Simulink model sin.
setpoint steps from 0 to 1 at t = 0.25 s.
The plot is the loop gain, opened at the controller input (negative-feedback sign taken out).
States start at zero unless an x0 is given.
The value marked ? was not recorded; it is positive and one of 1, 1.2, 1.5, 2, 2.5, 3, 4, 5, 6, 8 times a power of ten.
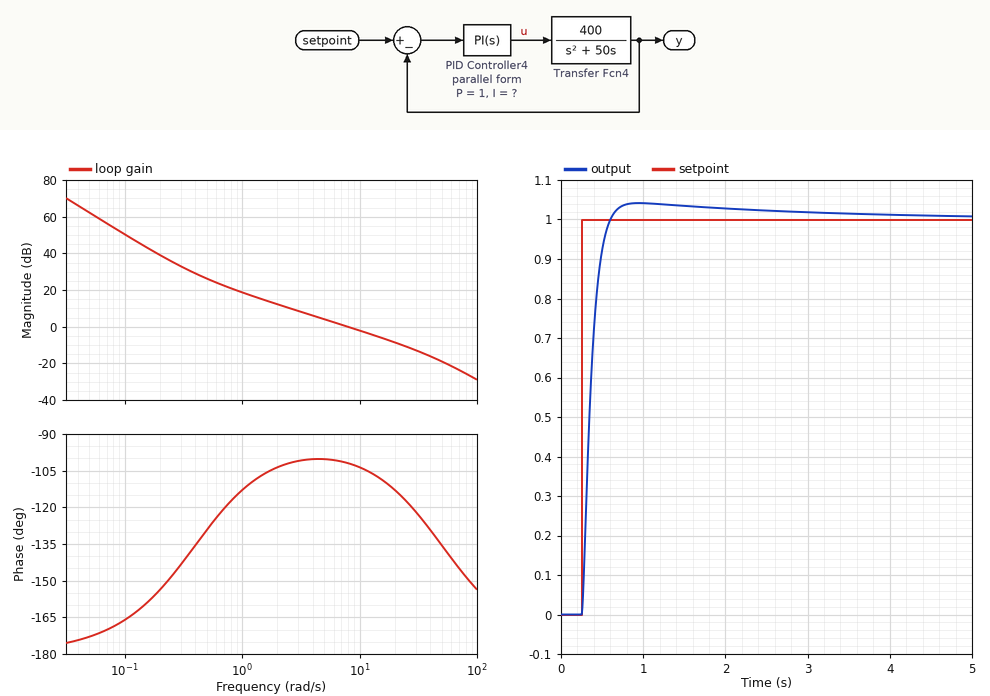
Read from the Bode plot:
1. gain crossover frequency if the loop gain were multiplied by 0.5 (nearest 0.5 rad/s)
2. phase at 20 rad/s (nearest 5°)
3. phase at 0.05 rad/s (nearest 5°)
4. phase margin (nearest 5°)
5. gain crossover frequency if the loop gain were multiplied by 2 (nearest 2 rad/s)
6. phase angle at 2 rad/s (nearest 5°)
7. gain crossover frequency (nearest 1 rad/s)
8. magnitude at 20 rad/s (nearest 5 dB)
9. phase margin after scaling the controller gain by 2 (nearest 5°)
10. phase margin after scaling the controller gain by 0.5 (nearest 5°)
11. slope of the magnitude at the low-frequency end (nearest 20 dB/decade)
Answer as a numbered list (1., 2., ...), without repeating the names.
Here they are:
1. 4.0 rad/s
2. -115°
3. -175°
4. 80°
5. 16 rad/s
6. -105°
7. 8 rad/s
8. -10 dB
9. 70°
10. 80°
11. -40 dB/decade
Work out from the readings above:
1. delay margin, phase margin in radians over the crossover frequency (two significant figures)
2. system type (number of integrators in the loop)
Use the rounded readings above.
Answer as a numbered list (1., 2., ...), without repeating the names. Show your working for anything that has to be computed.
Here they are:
1. 80 × π / 180 / 8 = 0.17 s
2. 2
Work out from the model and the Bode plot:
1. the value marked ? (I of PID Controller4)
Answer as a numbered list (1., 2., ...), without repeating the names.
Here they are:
1. 0.4
